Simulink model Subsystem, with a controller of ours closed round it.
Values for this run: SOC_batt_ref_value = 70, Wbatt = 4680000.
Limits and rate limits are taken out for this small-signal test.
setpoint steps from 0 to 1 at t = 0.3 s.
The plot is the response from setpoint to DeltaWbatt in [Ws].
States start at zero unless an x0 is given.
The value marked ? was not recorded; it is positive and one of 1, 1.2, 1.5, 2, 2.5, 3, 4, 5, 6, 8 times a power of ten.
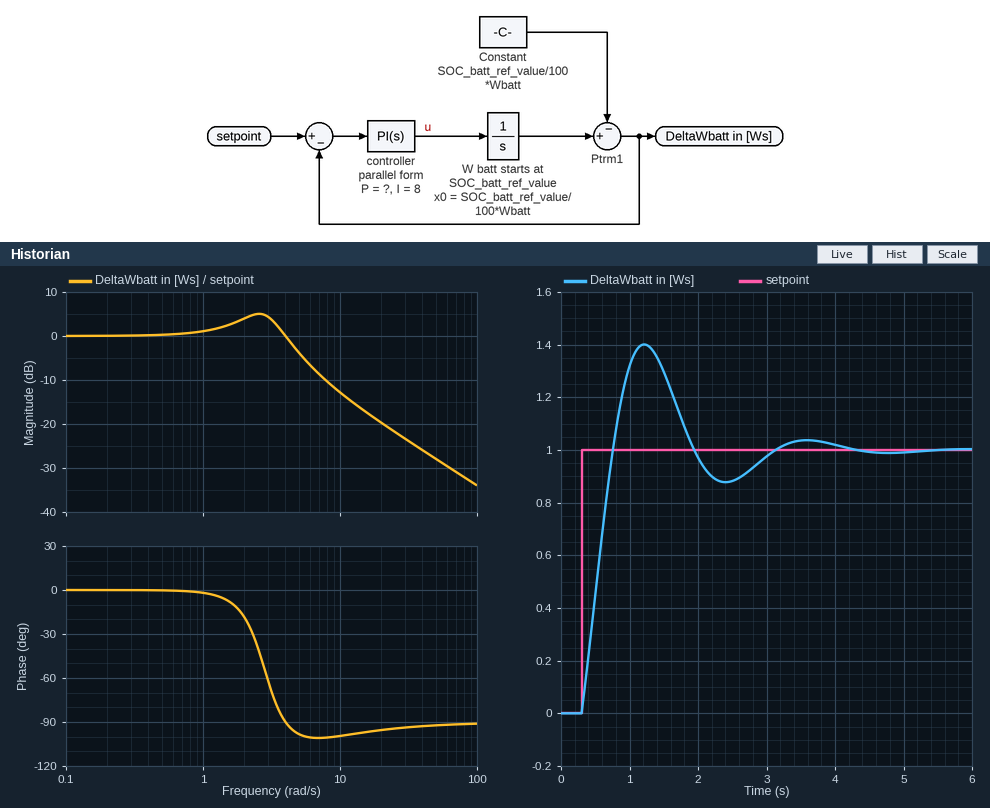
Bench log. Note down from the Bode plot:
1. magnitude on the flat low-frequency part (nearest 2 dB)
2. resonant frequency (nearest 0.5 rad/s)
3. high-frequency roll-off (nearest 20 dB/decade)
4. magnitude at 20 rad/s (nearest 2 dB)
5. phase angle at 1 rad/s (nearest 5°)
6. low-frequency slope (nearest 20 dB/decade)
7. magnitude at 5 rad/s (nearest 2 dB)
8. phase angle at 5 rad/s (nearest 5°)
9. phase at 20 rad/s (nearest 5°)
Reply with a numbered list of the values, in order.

1. 0 dB
2. 2.5 rad/s
3. -20 dB/decade
4. -20 dB
5. 0°
6. 0 dB/decade
7. -4 dB
8. -100°
9. -95°
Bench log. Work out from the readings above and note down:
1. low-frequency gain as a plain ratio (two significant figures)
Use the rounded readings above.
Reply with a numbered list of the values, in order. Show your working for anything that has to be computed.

1. 10^(0 / 20) = 1.0
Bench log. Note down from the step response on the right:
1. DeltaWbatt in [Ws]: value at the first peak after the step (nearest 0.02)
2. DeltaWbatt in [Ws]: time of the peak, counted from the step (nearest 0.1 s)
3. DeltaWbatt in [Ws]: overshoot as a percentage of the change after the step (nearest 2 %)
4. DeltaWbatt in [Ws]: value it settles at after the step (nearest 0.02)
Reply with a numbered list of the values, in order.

1. 1.40
2. 0.9 s
3. 40 %
4. 1.00
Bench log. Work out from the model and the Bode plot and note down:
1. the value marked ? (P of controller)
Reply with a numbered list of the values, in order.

1. 2
